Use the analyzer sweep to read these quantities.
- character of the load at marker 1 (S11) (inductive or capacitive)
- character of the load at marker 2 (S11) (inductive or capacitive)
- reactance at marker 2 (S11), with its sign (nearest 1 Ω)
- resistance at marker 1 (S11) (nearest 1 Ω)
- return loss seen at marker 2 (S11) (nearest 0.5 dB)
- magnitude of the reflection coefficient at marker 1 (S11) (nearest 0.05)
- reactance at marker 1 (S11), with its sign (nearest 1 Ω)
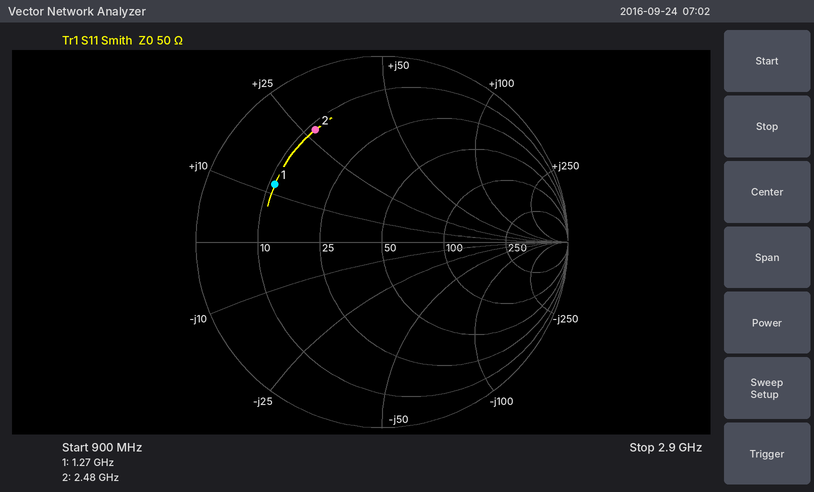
inductive
inductive
+27 Ω
11 Ω
3.0 dB
0.65
+12 Ω
